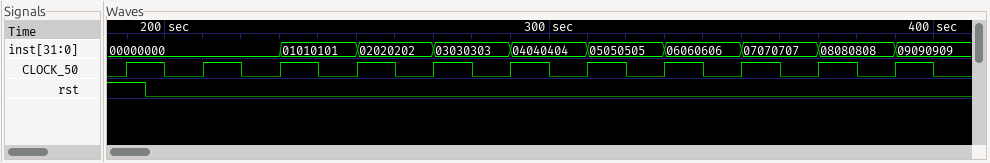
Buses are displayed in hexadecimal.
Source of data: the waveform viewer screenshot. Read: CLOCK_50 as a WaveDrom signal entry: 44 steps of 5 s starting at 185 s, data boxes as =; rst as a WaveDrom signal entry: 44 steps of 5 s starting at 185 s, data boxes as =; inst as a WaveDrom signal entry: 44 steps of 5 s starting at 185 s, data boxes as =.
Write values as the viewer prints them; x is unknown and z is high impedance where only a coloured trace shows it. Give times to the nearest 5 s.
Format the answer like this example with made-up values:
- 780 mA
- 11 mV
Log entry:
- {name: 'CLOCK_50', wave: '01.0.1.0.1.0.1.0.1.0.1.0.1.0.1.0.1.0.1.0.1.0'}
- {name: 'rst', wave: '1.0.........................................'}
- {name: 'inst', wave: '=........=...=...=...=...=...=...=...=...=..', data: '00000000 01010101 02020202 03030303 04040404 05050505 06060606 07070707 08080808 09090909'}
